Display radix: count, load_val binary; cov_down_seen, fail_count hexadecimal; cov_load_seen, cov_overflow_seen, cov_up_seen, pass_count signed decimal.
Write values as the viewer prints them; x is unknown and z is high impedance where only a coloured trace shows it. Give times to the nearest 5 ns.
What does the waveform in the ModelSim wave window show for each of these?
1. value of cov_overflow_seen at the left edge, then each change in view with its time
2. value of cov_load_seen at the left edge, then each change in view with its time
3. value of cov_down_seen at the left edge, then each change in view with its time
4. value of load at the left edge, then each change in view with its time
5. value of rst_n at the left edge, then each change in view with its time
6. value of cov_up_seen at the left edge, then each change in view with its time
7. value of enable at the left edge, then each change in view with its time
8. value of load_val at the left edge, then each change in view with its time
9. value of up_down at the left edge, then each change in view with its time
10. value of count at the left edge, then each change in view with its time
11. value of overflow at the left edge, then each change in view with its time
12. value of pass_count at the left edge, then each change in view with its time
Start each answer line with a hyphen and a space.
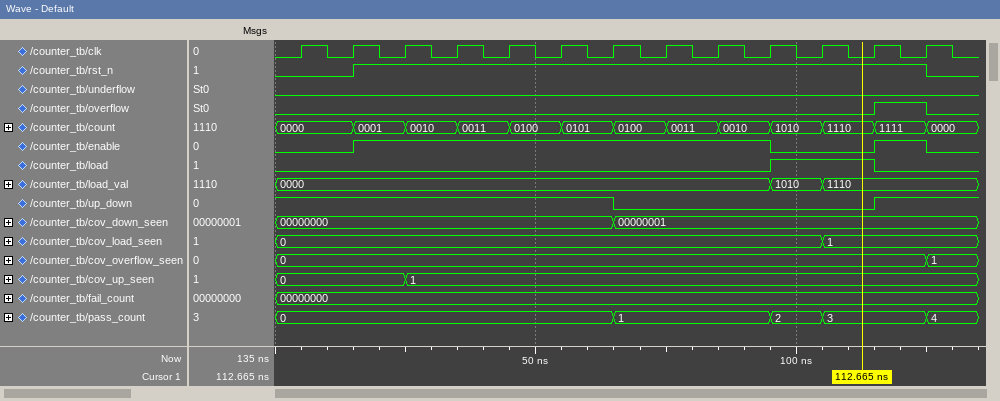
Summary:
- 0, 1 at 125 ns
- 0, 1 at 105 ns
- 00000000, 00000001 at 65 ns
- 0, 1 at 95 ns, 0 at 115 ns
- 0, 1 at 15 ns, 0 at 125 ns
- 0, 1 at 25 ns
- 0, 1 at 15 ns, 0 at 95 ns, 1 at 115 ns, 0 at 125 ns
- 0000, 1010 at 95 ns, 1110 at 105 ns
- 1, 0 at 65 ns, 1 at 115 ns
- 0000, 0001 at 15 ns, 0010 at 25 ns, 0011 at 35 ns, 0100 at 45 ns, 0101 at 55 ns, 0100 at 65 ns, 0011 at 75 ns, 0010 at 85 ns, 1010 at 95 ns, 1110 at 105 ns, 1111 at 115 ns, 0000 at 125 ns
- 0, 1 at 115 ns, 0 at 125 ns
- 0, 1 at 65 ns, 2 at 95 ns, 3 at 105 ns, 4 at 125 ns
